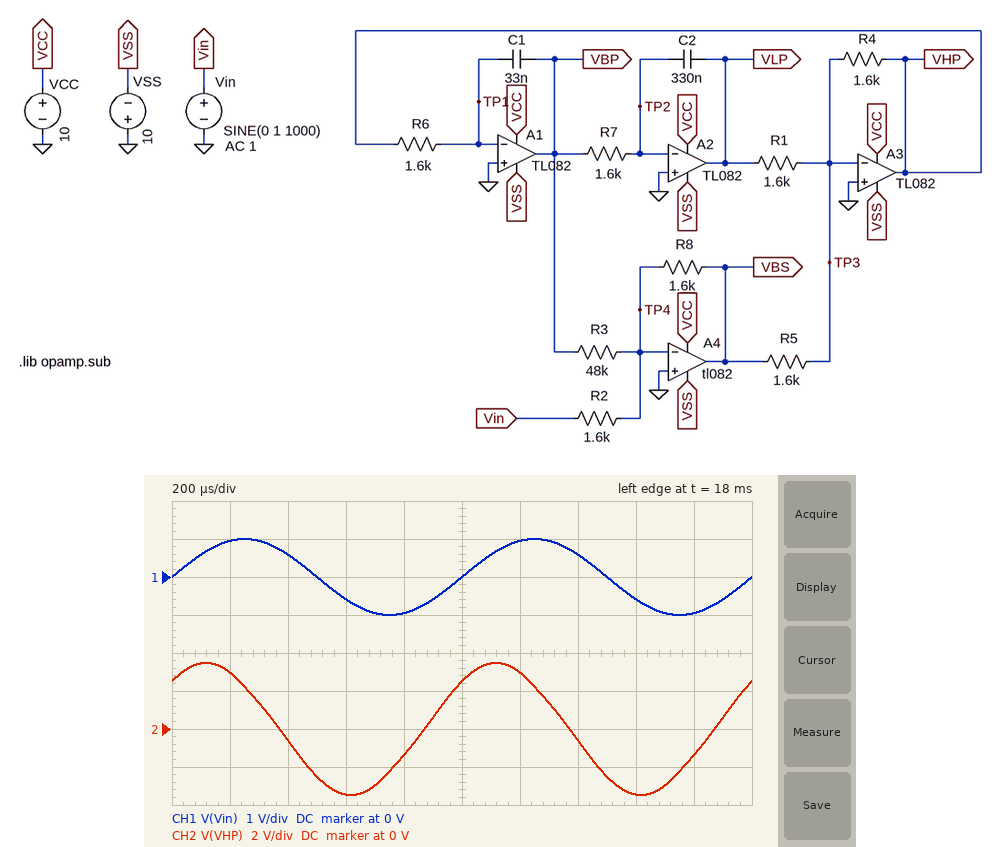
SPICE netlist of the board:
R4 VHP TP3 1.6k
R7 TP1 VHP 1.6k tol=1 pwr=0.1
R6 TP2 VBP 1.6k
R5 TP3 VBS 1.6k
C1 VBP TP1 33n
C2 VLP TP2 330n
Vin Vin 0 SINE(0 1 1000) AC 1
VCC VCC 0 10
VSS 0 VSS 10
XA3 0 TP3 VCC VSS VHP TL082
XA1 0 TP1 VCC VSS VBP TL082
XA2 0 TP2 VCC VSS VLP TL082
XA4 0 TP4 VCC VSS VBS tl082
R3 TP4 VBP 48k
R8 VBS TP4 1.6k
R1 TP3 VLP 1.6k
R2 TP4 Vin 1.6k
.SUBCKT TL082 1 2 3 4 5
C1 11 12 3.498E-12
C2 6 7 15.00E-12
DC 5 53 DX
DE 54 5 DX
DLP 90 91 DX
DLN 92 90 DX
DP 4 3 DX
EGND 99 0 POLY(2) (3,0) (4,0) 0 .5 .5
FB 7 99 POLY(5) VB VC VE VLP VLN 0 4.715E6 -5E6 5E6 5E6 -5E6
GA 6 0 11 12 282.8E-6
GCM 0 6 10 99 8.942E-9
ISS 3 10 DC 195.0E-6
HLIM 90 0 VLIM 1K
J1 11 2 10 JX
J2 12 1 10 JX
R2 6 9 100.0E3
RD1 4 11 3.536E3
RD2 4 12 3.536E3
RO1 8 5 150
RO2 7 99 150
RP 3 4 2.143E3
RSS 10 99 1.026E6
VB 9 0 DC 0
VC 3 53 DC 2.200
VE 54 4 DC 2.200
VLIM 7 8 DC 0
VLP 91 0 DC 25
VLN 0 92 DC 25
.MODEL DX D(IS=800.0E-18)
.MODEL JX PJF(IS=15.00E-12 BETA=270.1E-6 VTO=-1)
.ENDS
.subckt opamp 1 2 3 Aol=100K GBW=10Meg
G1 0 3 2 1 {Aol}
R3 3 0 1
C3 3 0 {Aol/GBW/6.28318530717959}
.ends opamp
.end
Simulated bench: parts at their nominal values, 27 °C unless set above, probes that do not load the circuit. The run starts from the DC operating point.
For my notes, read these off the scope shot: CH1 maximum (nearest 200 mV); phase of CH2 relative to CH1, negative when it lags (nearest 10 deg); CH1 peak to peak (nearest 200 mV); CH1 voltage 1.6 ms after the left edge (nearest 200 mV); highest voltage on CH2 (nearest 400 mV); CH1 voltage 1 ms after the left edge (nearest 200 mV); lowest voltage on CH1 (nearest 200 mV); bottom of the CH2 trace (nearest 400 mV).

1.0 V
50 deg
2.0 V
-600 mV
3.6 V
0 V
-1.0 V
-3.6 V
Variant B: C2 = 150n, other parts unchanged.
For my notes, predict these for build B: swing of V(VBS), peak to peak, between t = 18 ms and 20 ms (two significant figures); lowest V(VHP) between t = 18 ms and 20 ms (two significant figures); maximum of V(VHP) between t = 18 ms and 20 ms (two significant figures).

2.0 V
-1.0 V
1.0 V
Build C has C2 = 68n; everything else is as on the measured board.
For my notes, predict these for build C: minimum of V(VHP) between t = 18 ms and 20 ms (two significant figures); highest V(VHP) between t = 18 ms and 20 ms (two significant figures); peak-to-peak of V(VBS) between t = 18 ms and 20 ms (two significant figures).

-290 mV
300 mV
2.0 V
